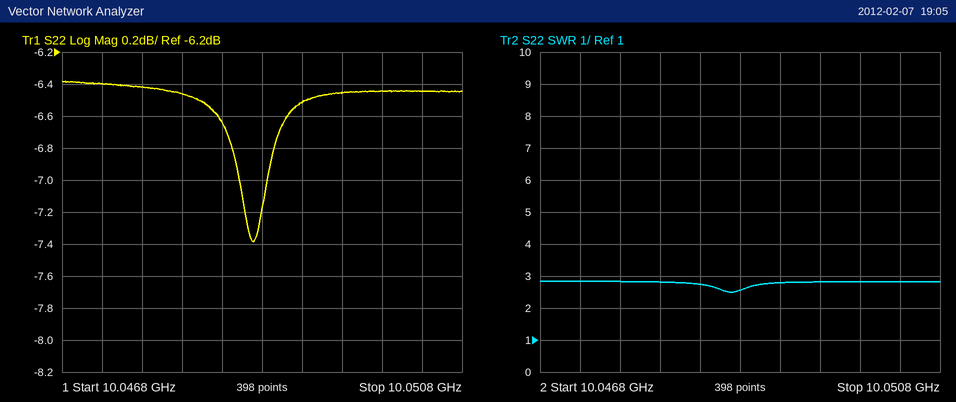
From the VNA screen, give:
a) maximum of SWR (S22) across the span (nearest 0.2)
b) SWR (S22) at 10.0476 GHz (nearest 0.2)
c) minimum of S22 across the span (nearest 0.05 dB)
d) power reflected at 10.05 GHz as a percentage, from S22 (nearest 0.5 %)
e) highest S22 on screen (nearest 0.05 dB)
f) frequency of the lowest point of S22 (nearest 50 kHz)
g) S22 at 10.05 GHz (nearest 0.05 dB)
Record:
2.8
2.8
-7.40 dB
22.5 %
-6.40 dB
10.04870 GHz
-6.45 dB
